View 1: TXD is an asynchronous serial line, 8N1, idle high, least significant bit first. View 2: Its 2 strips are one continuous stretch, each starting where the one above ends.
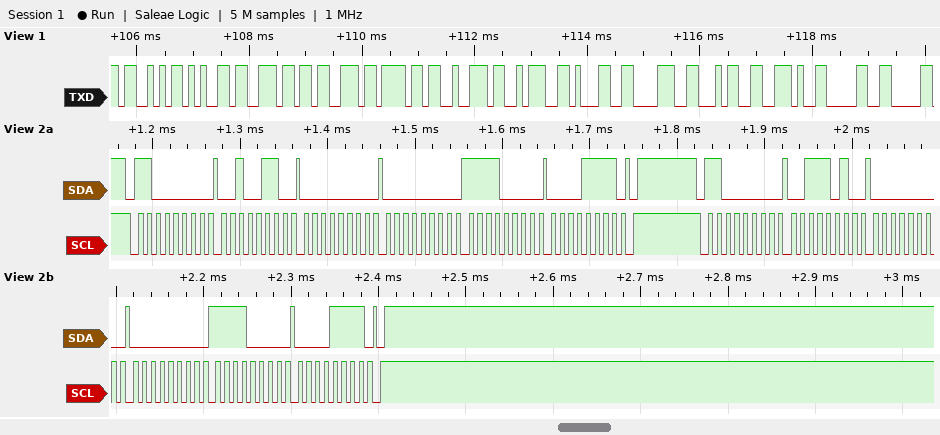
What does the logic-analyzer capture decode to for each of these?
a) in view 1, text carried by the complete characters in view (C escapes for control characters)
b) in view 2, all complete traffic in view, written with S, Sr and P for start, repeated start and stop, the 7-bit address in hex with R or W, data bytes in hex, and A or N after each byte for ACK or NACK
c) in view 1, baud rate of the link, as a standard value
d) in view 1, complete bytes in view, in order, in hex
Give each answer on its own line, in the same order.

"Sensor:184.0"
S 60W A 26 A 00 A 00 A F0 A 0F A P S 60W A 3A A 00 A 00 A F0 A 0F A P
9600 baud
53 65 6E 73 6F 72 3A 31 38 34 2E 30
